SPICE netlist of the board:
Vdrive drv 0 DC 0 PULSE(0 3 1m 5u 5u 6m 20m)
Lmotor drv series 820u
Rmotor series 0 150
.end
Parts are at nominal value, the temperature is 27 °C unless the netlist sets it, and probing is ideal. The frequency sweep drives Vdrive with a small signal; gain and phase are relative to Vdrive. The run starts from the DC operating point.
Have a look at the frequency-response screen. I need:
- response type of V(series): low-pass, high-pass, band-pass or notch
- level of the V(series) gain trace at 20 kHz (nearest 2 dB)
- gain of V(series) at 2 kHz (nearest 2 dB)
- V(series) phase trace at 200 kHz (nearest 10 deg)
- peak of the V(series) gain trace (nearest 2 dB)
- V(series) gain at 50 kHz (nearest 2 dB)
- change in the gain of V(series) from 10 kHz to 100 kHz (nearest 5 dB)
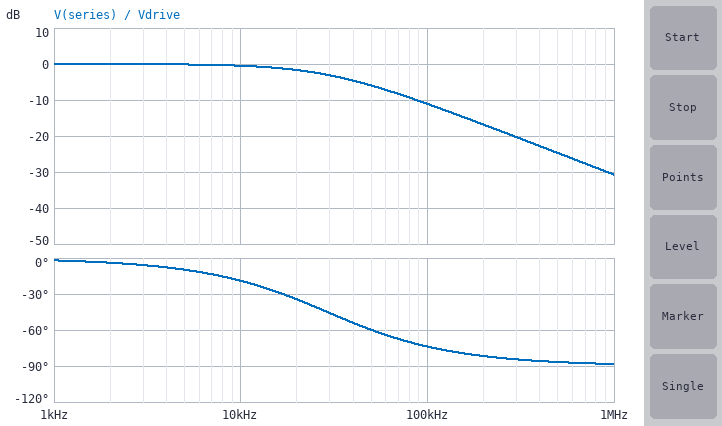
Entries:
low-pass
-2 dB
0 dB
-80 deg
0 dB
-6 dB
-10 dB
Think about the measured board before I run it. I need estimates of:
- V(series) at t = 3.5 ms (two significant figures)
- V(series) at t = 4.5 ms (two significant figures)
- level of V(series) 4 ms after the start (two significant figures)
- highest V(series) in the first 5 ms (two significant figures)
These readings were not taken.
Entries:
3.0 V
3.0 V
3.0 V
3.0 V
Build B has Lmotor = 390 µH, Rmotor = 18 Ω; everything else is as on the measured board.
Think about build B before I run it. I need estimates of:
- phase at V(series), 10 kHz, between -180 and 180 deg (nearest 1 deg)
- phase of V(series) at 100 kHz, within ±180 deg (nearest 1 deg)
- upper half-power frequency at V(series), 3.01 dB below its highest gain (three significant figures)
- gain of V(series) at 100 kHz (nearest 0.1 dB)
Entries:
-54 deg
-86 deg
7.35 kHz
-22.7 dB
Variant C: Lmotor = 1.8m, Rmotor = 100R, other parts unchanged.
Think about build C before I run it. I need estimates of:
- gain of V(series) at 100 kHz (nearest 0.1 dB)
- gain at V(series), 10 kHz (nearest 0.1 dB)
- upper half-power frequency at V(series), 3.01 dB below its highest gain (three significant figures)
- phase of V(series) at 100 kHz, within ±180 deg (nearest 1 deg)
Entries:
-21.1 dB
-3.6 dB
8.84 kHz
-85 deg
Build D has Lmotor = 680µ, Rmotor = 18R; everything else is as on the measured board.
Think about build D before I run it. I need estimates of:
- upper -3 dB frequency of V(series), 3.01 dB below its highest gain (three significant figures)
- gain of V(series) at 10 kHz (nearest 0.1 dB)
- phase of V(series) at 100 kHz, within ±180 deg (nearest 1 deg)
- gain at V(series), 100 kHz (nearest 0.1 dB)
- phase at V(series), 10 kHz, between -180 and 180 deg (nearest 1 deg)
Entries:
4.21 kHz
-8.2 dB
-88 deg
-27.5 dB
-67 deg
